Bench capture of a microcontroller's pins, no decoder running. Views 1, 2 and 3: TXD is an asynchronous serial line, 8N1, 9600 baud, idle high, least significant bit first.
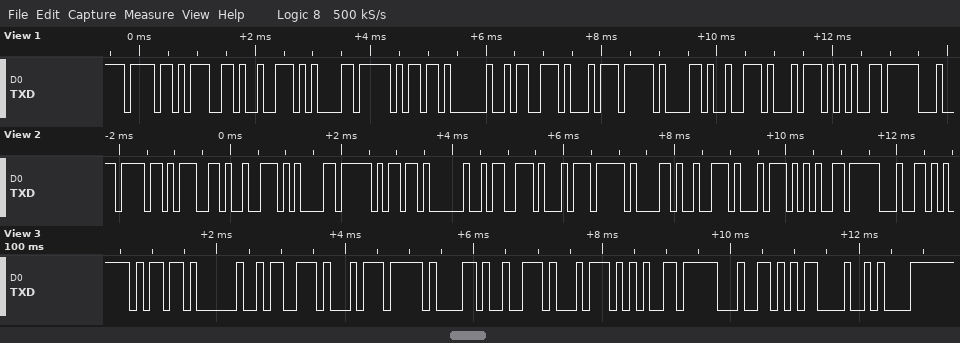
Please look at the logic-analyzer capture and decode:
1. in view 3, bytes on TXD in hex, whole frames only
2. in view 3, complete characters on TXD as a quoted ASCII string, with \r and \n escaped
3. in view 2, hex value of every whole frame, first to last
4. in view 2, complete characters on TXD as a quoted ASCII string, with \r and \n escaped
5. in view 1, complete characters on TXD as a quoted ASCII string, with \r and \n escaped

6D 20 73 74 61 72 74 65 64 0D 0A
"m started\r\n"
6F 67 72 61 6D 20 73 74 61 72 74 65 64
"ogram started"
"ogram starte"
